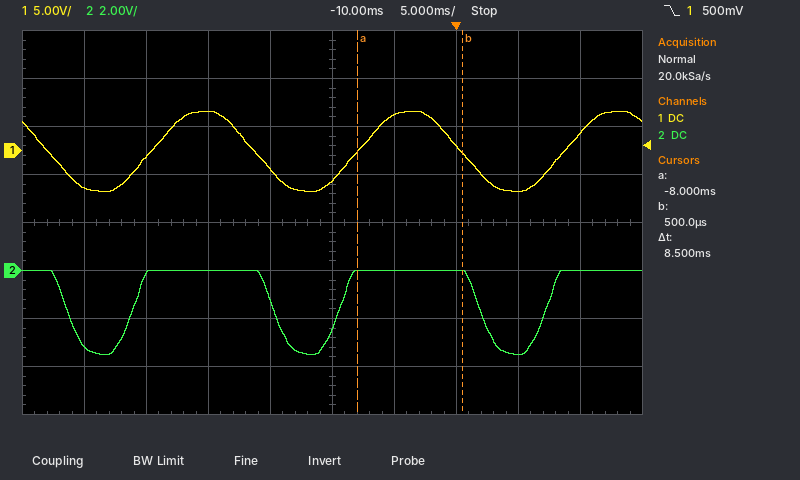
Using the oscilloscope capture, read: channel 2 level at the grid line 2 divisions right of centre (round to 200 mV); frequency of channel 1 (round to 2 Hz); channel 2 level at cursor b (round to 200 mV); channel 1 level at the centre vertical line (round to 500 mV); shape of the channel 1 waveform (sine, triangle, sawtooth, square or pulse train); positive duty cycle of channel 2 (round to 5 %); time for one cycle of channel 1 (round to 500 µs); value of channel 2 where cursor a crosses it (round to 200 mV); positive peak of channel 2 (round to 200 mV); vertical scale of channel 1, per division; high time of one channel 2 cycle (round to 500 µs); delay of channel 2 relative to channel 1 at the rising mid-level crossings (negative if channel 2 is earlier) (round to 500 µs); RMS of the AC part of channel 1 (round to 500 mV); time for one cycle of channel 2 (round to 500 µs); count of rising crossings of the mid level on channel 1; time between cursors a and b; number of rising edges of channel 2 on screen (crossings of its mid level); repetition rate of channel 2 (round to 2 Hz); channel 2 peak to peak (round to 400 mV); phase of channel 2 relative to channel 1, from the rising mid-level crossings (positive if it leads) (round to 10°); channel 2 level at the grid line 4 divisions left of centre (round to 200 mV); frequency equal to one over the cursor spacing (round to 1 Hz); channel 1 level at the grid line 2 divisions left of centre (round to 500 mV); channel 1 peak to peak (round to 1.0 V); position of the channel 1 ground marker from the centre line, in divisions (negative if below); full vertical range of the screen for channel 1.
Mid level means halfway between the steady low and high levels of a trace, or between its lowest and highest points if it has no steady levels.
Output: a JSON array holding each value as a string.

["0.0 V", "60 Hz", "0.0 V", "-3.0 V", "sine", "70 %", "16.5 ms", "0.0 V", "0.0 V", "5 V", "11.5 ms", "-1.5 ms", "3.0 V", "16.5 ms", "3", "8.5 ms", "3", "60 Hz", "3.6 V", "+30°", "-3.2 V", "118 Hz", "4.0 V", "8.0 V", "+1.5 div", "40 V"]
